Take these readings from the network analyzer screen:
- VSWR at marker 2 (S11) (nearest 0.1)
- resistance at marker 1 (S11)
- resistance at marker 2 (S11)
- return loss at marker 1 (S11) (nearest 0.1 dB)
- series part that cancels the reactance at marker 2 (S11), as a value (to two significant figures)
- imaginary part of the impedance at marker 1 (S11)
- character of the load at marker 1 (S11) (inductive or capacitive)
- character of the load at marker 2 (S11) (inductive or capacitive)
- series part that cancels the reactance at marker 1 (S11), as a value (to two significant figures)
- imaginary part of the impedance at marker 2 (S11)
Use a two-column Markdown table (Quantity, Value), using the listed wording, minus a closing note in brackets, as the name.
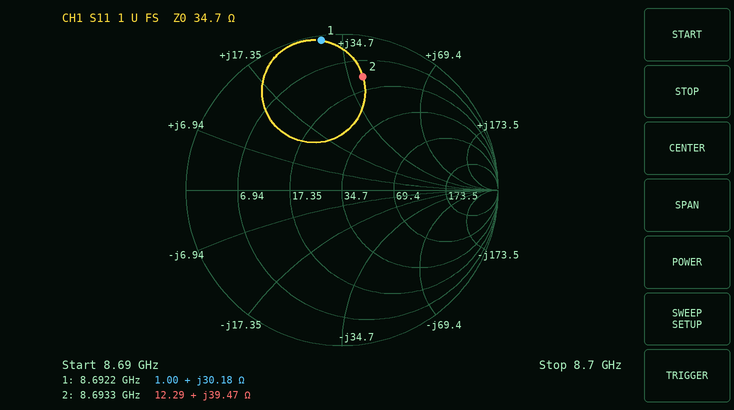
| Quantity | Value |
|---|---|
| VSWR at marker 2 (S11) | 6.7 |
| resistance at marker 1 | 1.00 Ω |
| resistance at marker 2 | 12.29 Ω |
| return loss at marker 1 (S11) | 0.3 dB |
| series part that cancels the reactance at marker 2 (S11), as a value | 460 fF |
| imaginary part of the impedance at marker 1 | +30.18 Ω |
| character of the load at marker 1 (S11) | inductive |
| character of the load at marker 2 (S11) | inductive |
| series part that cancels the reactance at marker 1 (S11), as a value | 610 fF |
| imaginary part of the impedance at marker 2 | +39.47 Ω |
